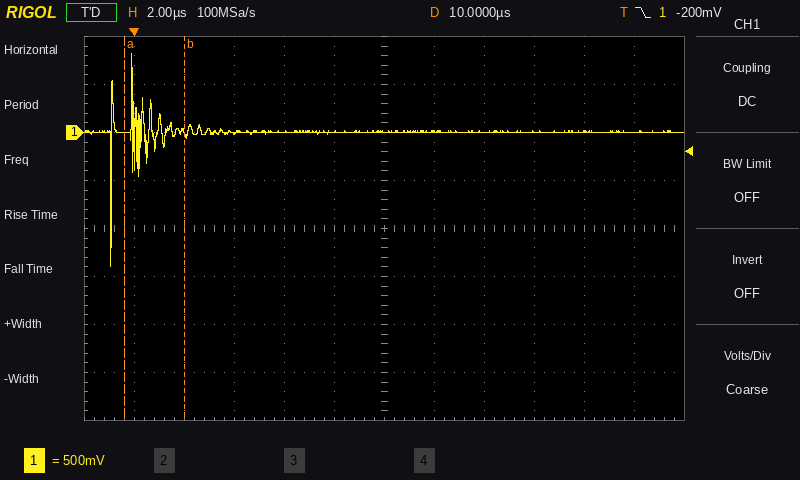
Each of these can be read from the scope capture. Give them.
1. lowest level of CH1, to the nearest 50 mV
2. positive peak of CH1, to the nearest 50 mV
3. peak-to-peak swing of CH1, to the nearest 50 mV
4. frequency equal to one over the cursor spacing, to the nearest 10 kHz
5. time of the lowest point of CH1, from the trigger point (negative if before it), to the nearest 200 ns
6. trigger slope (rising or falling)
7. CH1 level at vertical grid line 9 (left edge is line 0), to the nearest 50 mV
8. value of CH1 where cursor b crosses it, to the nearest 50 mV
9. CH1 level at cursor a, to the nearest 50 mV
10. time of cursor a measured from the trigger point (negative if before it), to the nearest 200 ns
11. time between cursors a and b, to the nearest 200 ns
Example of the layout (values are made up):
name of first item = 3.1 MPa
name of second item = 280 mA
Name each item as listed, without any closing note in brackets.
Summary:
lowest level of CH1, to the nearest 50 mV = -1.40 V
positive peak of CH1, to the nearest 50 mV = 800 mV
peak-to-peak swing of CH1, to the nearest 50 mV = 2.20 V
frequency equal to one over the cursor spacing, to the nearest 10 kHz = 420 kHz
time of the lowest point of CH1, from the trigger point (negative if before it), to the nearest 200 ns = -1.0 µs
trigger slope = falling
CH1 level at vertical grid line 9 (left edge is line 0), to the nearest 50 mV = 0 mV
value of CH1 where cursor b crosses it, to the nearest 50 mV = 0 mV
CH1 level at cursor a, to the nearest 50 mV = 0 mV
time of cursor a measured from the trigger point (negative if before it), to the nearest 200 ns = -400 ns
time between cursors a and b, to the nearest 200 ns = 2.4 µs
